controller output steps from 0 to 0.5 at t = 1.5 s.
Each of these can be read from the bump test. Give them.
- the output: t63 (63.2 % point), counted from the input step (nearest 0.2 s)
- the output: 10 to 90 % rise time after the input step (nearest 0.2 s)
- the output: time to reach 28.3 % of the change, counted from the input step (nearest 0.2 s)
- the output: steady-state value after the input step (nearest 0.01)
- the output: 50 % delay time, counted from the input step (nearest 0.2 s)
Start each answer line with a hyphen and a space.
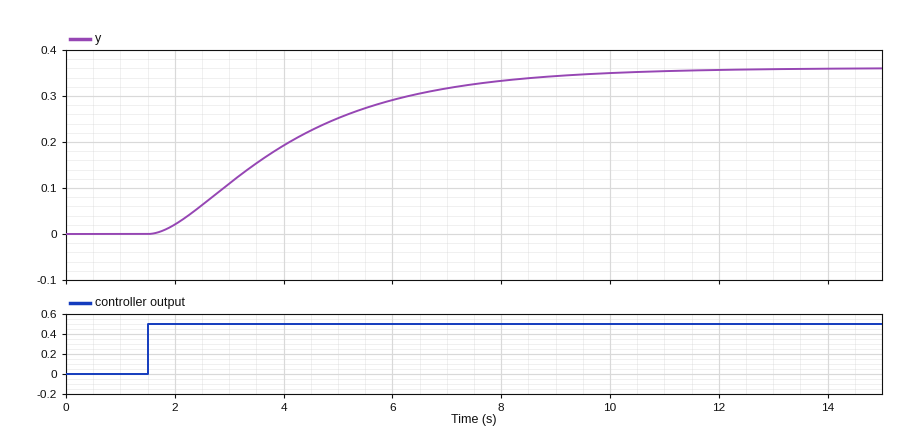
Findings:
- 3.0 s
- 5.2 s
- 1.4 s
- 0.36
- 2.4 s
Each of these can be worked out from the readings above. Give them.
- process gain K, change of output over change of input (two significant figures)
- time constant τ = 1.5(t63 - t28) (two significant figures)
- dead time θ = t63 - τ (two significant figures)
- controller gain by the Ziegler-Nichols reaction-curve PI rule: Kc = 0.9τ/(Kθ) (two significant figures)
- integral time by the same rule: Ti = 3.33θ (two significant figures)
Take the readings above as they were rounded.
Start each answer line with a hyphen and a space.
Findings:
- 0.72
- 2.4 s
- 0.60 s
- 5.0
- 2.0 s
